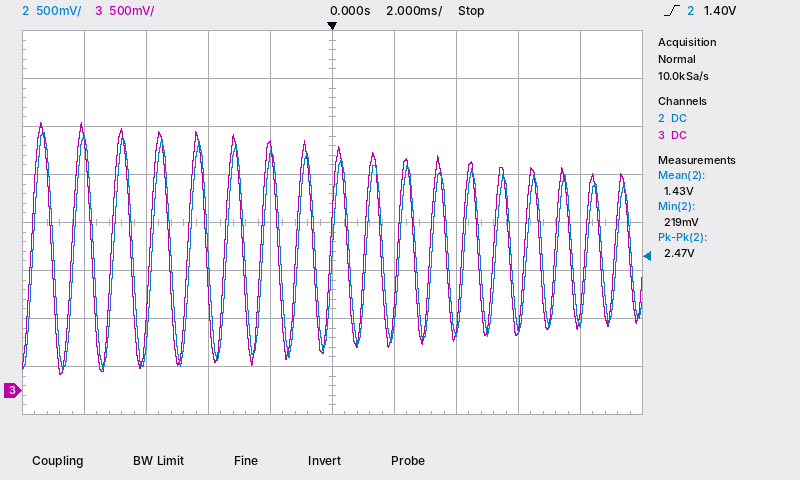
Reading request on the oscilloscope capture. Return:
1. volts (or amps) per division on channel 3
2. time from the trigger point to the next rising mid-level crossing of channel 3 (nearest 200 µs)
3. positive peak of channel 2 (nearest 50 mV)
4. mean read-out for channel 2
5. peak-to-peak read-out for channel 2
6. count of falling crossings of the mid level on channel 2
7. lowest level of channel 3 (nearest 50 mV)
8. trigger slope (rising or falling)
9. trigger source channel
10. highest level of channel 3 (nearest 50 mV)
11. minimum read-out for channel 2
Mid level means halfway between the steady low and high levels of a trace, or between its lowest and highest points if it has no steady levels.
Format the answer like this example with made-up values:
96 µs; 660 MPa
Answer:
500 mV; 1.0 ms; 2.70 V; 1.43 V; 2.47 V; 18; 150 mV; rising; channel 2; 2.80 V; 219 mV
